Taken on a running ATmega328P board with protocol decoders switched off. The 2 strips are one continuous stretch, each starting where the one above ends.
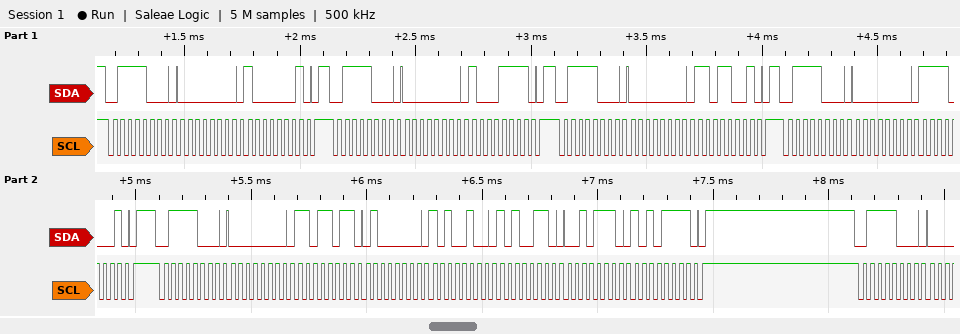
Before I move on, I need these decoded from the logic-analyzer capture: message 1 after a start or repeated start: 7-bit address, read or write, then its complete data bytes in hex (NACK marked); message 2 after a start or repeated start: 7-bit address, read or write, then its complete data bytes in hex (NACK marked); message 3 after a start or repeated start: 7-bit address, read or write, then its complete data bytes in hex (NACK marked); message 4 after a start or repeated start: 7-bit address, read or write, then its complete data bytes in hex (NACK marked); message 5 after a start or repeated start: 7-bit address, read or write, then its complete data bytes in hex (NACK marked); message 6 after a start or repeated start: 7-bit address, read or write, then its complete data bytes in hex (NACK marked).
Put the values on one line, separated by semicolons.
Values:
0x3C write: 00 81; 0x3C write: 00 8F; 0x3C write: 00 D9; 0x3C write: 00 F1; 0x3C write: 00 DB 40 A4 A6 2E AF; 0x3C write
